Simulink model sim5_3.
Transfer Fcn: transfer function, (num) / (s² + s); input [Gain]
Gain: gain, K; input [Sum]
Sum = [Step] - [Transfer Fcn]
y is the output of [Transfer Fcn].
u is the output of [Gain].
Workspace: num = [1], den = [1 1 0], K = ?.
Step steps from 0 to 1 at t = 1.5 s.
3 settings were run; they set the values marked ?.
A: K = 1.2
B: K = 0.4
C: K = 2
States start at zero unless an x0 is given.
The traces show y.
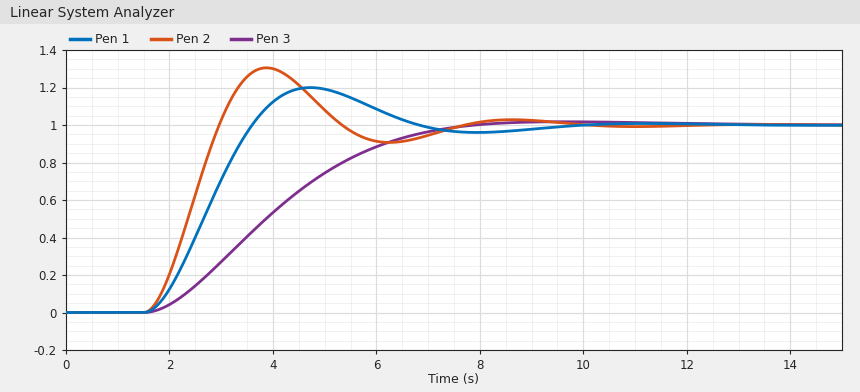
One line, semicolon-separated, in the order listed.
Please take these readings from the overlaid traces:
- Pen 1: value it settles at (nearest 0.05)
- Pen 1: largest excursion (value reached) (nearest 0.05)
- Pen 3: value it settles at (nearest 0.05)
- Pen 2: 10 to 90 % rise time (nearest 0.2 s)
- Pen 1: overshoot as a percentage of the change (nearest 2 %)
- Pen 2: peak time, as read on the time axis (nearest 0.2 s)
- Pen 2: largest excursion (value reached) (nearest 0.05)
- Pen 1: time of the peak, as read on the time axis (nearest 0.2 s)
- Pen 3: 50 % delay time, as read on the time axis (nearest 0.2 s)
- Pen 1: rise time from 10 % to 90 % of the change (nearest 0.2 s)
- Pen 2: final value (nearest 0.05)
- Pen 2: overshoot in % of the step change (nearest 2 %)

1.00; 1.20; 1.00; 1.0 s; 20 %; 3.8 s; 1.30; 4.8 s; 3.8 s; 1.4 s; 1.00; 30 %
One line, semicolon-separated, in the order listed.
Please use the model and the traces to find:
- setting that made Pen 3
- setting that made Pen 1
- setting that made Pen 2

B; A; C
